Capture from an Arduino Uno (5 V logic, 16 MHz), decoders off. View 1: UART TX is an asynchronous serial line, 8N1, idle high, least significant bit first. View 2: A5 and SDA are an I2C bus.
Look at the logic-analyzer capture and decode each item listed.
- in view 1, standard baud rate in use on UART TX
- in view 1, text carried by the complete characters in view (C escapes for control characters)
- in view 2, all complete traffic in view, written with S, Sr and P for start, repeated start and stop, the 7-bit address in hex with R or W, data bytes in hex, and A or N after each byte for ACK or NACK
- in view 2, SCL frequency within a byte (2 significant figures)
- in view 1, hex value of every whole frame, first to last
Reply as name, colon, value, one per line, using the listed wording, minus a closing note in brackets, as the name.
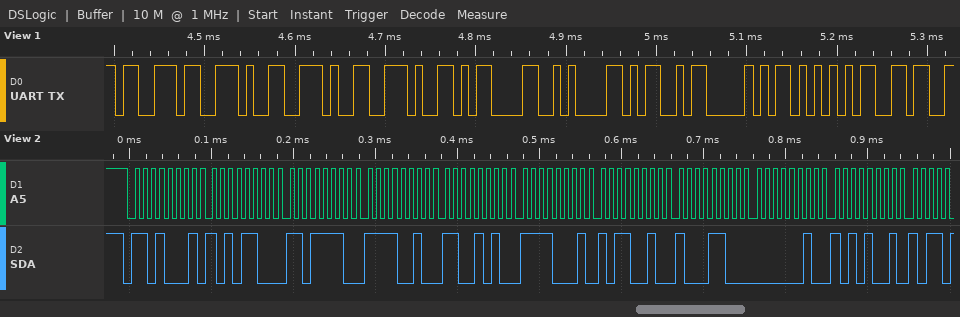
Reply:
in view 1, standard baud rate in use on UART TX: 115200 baud
in view 1, text carried by the complete characters in view: "s...\r\nMPU6"
in view 2, all complete traffic in view, written with S, Sr and P for start, repeated start and stop, the 7-bit address in hex with R or W, data bytes in hex, and A or N after each byte for ACK or NACK: S 68R A AC A DE A F2 A CA A F1 A B2 A 8C A 02 A A9 A
in view 2, SCL frequency within a byte: 100 kHz
in view 1, hex value of every whole frame, first to last: 73 2E 2E 2E 0D 0A 4D 50 55 36
